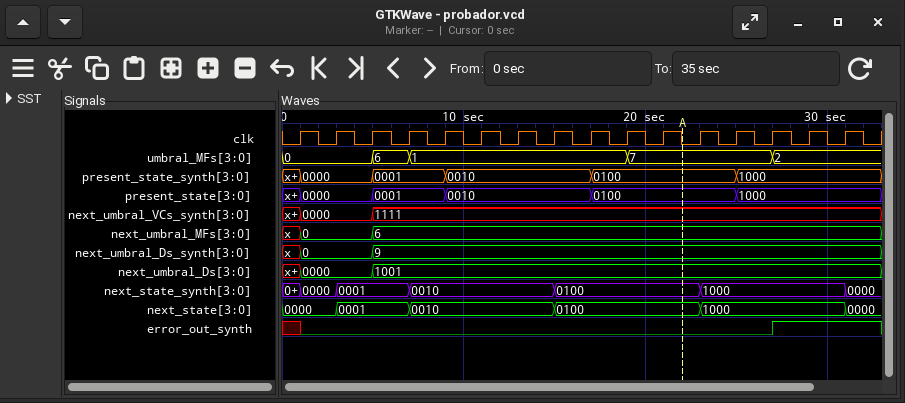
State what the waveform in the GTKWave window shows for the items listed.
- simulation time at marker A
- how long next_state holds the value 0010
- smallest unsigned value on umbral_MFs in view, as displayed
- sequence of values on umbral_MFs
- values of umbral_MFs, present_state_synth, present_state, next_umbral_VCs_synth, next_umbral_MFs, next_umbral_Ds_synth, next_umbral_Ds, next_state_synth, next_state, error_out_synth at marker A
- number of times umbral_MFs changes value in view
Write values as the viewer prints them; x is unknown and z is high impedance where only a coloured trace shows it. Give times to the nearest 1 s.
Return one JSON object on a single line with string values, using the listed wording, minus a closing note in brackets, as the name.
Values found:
{"simulation time at marker A": "22 s", "how long next_state holds the value 0010": "8 s", "smallest unsigned value on umbral_MFs in view, as displayed": "0", "sequence of values on umbral_MFs": "0, 6, 1, 7, 2", "values of umbral_MFs, present_state_synth, present_state, next_umbral_VCs_synth, next_umbral_MFs, next_umbral_Ds_synth, next_umbral_Ds, next_state_synth, next_state, error_out_synth at marker A": "umbral_MFs=7, present_state_synth=0100, present_state=0100, next_umbral_VCs_synth=1111, next_umbral_MFs=6, next_umbral_Ds_synth=9, next_umbral_Ds=1001, next_state_synth=0100, next_state=0100, error_out_synth=0", "number of times umbral_MFs changes value in view": "4"}
